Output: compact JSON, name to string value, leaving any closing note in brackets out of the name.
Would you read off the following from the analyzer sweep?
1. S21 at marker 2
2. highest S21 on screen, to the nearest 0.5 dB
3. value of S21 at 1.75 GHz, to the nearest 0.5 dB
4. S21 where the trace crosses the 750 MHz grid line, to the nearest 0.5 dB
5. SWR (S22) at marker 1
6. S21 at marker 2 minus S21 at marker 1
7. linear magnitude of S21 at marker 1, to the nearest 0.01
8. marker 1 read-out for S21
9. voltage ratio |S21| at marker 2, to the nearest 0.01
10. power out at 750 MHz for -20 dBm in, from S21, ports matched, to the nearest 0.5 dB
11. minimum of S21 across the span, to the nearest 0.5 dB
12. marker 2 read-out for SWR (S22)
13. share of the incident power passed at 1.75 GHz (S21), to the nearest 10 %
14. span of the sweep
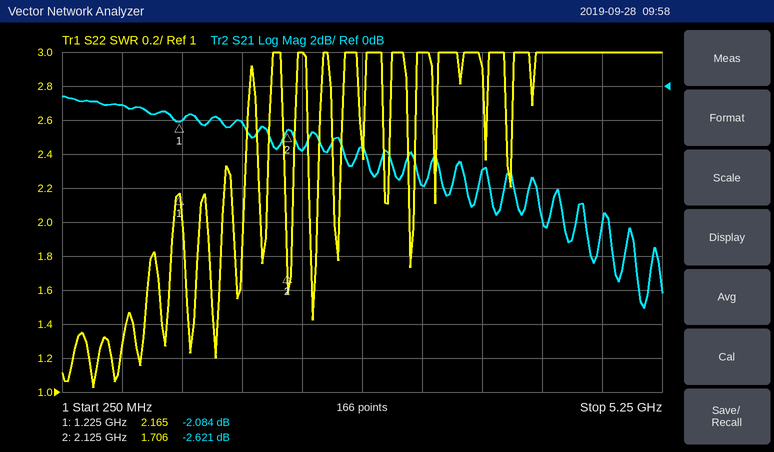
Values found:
{"S21 at marker 2": "-2.621 dB", "highest S21 on screen, to the nearest 0.5 dB": "-0.5 dB", "value of S21 at 1.75 GHz, to the nearest 0.5 dB": "-2.0 dB", "S21 where the trace crosses the 750 MHz grid line, to the nearest 0.5 dB": "-1.0 dB", "SWR (S22) at marker 1": "2.165", "S21 at marker 2 minus S21 at marker 1": "-0.537 dB", "linear magnitude of S21 at marker 1, to the nearest 0.01": "0.79", "marker 1 read-out for S21": "-2.084 dB", "voltage ratio |S21| at marker 2, to the nearest 0.01": "0.74", "power out at 750 MHz for -20 dBm in, from S21, ports matched, to the nearest 0.5 dB": "-21.0 dBm", "minimum of S21 across the span, to the nearest 0.5 dB": "-13.0 dB", "marker 2 read-out for SWR": "1.706", "share of the incident power passed at 1.75 GHz (S21), to the nearest 10 %": "60 %", "span of the sweep": "5 GHz"}
